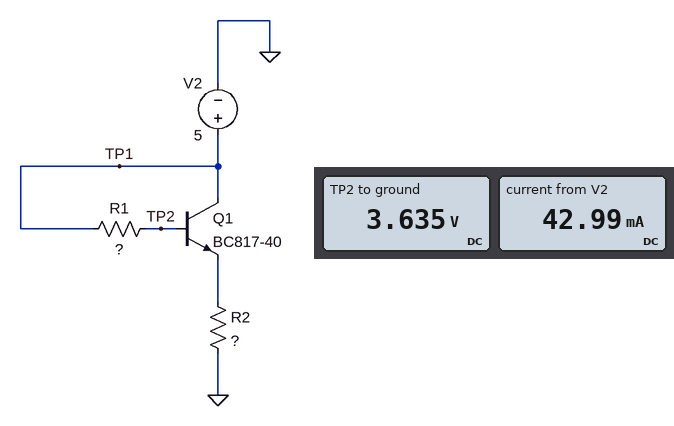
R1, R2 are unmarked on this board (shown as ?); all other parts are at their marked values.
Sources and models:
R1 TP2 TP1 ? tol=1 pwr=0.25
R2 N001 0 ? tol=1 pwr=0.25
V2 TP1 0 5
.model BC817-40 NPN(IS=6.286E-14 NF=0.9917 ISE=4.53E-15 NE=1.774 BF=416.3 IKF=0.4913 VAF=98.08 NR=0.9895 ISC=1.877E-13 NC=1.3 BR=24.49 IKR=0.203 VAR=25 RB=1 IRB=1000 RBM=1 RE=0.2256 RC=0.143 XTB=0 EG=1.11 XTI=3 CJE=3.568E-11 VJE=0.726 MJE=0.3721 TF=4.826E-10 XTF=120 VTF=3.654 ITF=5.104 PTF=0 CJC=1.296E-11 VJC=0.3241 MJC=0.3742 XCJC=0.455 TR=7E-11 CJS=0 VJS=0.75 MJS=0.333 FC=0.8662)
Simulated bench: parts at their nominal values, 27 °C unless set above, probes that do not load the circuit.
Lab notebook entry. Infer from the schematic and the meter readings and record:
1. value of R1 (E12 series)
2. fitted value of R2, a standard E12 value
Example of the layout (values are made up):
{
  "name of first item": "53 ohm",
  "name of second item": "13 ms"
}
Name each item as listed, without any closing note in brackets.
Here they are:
{
  "value of R1": "12 kΩ",
  "fitted value of R2, a standard E12 value": "68 Ω"
}
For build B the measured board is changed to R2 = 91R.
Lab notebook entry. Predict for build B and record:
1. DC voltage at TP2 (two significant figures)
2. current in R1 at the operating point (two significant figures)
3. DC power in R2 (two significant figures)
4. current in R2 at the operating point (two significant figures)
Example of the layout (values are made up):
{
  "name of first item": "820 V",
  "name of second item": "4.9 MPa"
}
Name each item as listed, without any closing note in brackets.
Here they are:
{
  "DC voltage at TP2": "3.9 V",
  "current in R1 at the operating point": "92 µA",
  "DC power in R2": "110 mW",
  "current in R2 at the operating point": "35 mA"
}
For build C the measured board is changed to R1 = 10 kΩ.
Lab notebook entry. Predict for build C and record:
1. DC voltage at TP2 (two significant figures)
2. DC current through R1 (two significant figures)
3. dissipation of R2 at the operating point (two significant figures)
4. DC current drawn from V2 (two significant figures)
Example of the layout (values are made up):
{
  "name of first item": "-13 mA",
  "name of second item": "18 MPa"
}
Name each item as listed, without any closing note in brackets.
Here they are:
{
  "DC voltage at TP2": "3.8 V",
  "DC current through R1": "120 µA",
  "dissipation of R2 at the operating point": "140 mW",
  "DC current drawn from V2": "45 mA"
}
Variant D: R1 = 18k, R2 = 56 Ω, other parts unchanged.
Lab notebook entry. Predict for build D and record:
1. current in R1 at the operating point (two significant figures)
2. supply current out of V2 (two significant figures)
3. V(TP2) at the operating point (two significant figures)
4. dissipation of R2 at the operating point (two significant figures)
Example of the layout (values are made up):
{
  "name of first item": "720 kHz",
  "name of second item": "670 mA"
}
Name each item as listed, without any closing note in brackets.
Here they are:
{
  "current in R1 at the operating point": "110 µA",
  "supply current out of V2": "42 mA",
  "V(TP2) at the operating point": "3.0 V",
  "dissipation of R2 at the operating point": "97 mW"
}
